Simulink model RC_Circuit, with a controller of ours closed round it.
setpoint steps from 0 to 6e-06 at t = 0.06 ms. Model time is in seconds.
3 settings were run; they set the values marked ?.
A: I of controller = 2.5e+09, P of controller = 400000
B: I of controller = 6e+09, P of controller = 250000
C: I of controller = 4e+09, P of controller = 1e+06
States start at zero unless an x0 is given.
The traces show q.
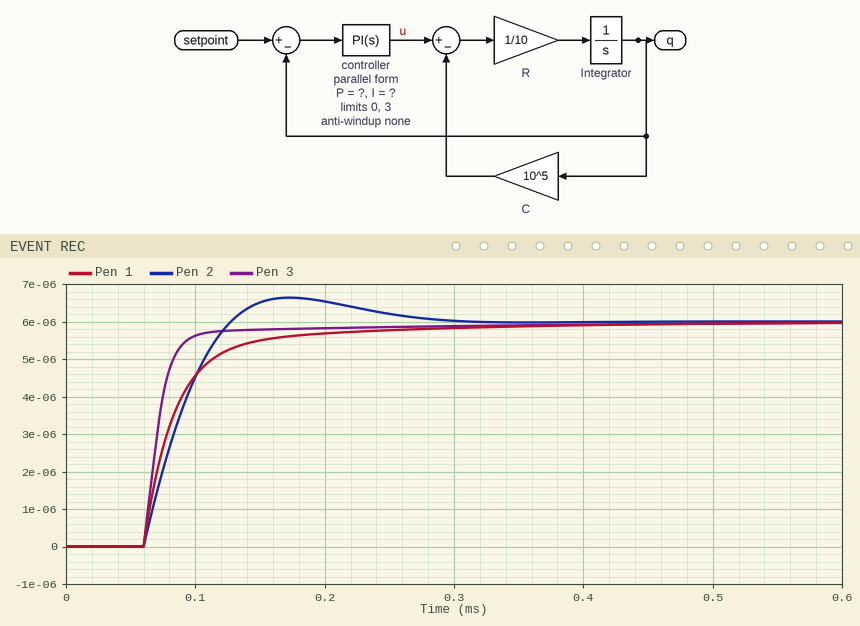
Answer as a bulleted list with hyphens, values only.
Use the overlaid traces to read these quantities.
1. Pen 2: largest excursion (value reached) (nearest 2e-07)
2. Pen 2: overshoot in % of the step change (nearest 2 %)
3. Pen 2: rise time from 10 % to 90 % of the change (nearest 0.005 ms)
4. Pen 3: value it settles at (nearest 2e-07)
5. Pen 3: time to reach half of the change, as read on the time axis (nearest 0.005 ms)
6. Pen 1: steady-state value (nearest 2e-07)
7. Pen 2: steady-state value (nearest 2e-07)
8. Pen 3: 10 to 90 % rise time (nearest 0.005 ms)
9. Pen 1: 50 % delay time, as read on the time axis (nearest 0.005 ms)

- 0.0000066
- 10 %
- 0.050 ms
- 0.0000060
- 0.070 ms
- 0.0000060
- 0.0000060
- 0.030 ms
- 0.080 ms
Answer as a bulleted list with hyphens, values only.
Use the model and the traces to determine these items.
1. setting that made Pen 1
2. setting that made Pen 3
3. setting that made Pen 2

- A
- C
- B
